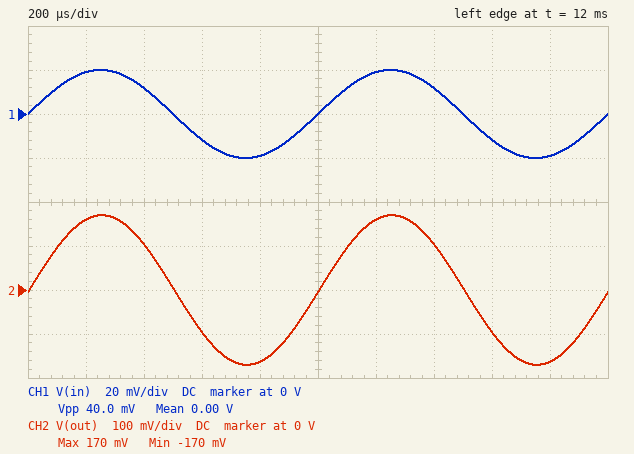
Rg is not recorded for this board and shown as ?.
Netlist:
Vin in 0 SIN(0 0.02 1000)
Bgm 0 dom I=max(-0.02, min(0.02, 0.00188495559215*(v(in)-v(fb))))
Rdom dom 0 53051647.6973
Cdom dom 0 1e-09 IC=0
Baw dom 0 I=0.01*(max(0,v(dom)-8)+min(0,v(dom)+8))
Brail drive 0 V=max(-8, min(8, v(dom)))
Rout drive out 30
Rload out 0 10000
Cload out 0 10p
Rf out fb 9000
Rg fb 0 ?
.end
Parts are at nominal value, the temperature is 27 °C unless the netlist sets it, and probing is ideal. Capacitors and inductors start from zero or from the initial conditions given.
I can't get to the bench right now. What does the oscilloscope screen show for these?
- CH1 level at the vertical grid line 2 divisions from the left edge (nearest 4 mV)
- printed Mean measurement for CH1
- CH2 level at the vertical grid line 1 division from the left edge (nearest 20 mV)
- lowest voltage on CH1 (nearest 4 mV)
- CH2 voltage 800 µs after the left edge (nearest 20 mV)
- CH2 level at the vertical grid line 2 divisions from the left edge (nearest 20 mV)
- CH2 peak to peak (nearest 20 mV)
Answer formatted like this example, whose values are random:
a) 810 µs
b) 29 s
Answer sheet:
a) 12 mV
b) 0.00 V
c) 160 mV
d) -20 mV
e) -160 mV
f) 100 mV
g) 340 mV
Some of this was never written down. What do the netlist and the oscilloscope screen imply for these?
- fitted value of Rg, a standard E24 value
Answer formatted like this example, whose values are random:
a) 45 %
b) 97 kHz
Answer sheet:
a) 1.2 kΩ
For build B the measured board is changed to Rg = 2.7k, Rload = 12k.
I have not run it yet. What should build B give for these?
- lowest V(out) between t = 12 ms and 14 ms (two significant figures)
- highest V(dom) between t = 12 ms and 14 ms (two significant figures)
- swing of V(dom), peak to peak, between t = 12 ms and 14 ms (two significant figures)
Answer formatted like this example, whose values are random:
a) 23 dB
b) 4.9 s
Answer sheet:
a) -87 mV
b) 87 mV
c) 170 mV
